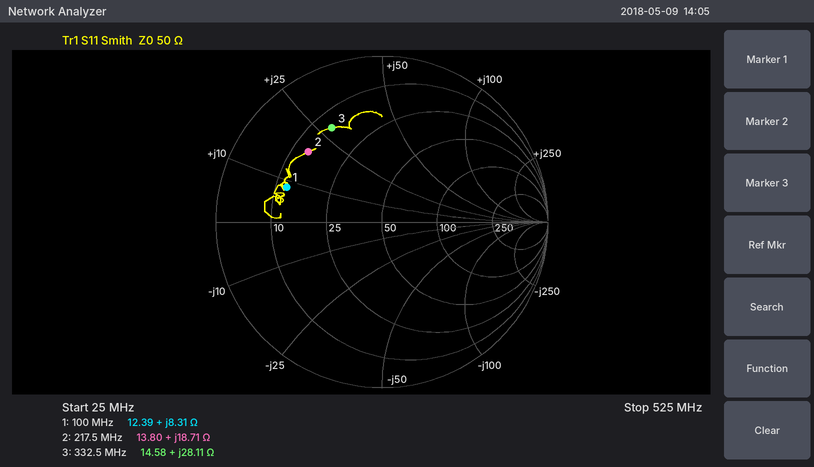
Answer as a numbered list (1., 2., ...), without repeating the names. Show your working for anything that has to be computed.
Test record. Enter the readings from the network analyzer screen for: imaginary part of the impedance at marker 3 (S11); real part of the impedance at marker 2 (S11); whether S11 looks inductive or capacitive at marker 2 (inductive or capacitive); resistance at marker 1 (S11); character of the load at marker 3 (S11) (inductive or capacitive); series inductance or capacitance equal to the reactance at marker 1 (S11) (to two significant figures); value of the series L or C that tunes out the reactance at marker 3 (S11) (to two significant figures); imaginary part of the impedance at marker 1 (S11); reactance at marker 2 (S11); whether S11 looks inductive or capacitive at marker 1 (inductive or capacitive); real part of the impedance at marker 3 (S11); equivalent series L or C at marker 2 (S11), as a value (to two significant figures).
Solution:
1. +28.11 Ω
2. 13.80 Ω
3. inductive
4. 12.39 Ω
5. inductive
6. L = 8.31 Ω/(2π × 100 MHz) ≈ 13 nH
7. C = 1/(2π × 332.5 MHz × 28.11 Ω) ≈ 17 pF
8. +8.31 Ω
9. +18.71 Ω
10. inductive
11. 14.58 Ω
12. L = 18.71 Ω/(2π × 217.5 MHz) ≈ 14 nH
